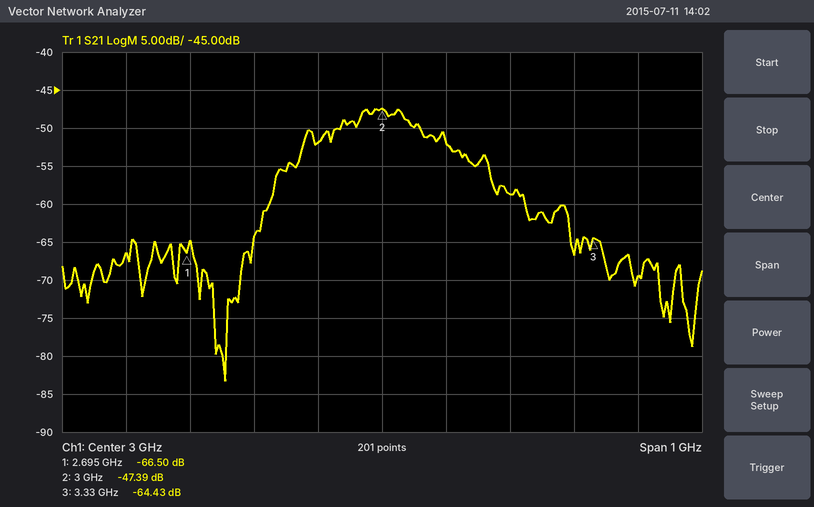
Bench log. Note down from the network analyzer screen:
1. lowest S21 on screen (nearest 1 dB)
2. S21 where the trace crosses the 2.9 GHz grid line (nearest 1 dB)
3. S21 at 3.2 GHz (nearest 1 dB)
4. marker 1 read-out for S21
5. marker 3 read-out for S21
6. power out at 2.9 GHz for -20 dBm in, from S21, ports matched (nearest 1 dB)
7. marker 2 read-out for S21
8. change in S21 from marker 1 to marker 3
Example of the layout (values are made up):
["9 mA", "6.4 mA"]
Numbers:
["-83 dB", "-52 dB", "-59 dB", "-66.50 dB", "-64.43 dB", "-72 dBm", "-47.39 dB", "2.07 dB"]
